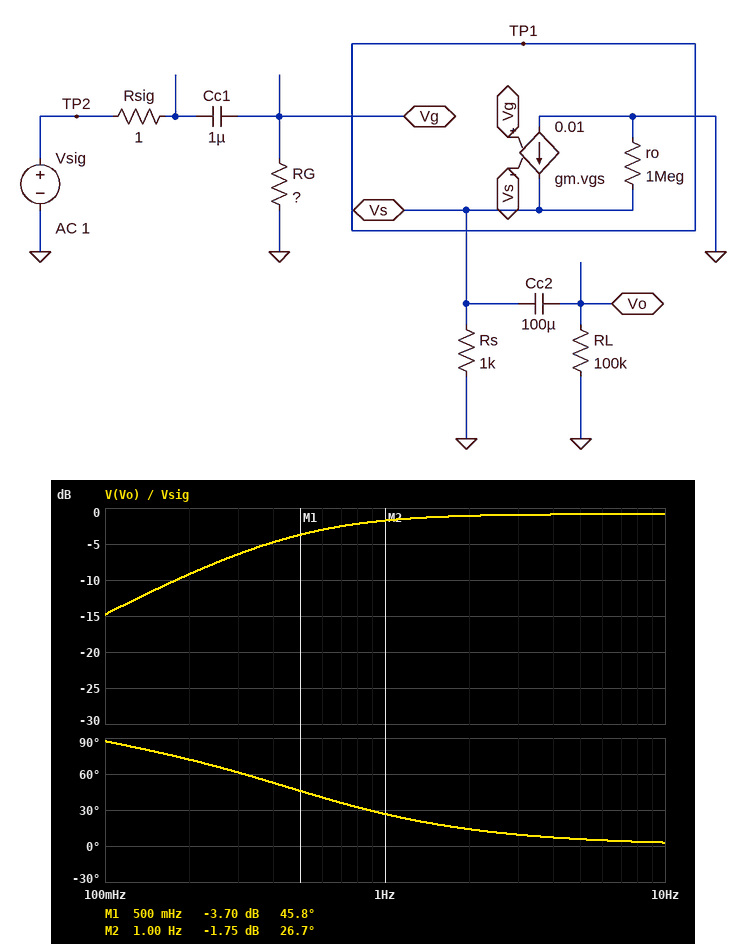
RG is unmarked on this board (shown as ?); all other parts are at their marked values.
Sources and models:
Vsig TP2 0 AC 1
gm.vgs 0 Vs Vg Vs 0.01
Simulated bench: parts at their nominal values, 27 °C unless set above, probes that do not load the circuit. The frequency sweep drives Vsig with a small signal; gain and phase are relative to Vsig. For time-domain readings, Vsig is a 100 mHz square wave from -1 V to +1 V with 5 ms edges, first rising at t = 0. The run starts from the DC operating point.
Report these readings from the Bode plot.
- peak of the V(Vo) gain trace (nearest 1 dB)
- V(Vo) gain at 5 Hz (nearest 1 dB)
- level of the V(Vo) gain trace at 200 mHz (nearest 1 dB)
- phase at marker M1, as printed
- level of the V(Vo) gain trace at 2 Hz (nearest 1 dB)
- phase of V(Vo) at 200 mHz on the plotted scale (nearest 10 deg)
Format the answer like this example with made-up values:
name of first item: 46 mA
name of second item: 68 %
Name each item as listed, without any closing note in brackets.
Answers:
peak of the V(Vo) gain trace: -1 dB
V(Vo) gain at 5 Hz: -1 dB
level of the V(Vo) gain trace at 200 mHz: -9 dB
phase at marker M1, as printed: 45.8 deg
level of the V(Vo) gain trace at 2 Hz: -1 dB
phase of V(Vo) at 200 mHz on the plotted scale: 70 deg
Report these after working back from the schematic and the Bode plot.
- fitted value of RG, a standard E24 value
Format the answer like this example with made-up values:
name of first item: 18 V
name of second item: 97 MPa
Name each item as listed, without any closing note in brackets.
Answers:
fitted value of RG, a standard E24 value: 330 kΩ
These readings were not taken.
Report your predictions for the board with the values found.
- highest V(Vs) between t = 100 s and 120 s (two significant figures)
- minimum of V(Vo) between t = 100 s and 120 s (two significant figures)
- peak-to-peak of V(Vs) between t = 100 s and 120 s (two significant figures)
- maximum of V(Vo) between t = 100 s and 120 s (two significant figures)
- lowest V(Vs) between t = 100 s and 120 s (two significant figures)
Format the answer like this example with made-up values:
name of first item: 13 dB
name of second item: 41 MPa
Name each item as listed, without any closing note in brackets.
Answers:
highest V(Vs) between t = 100 s and 120 s: 1.8 V
minimum of V(Vo) between t = 100 s and 120 s: -1.8 V
peak-to-peak of V(Vs) between t = 100 s and 120 s: 3.6 V
maximum of V(Vo) between t = 100 s and 120 s: 1.8 V
lowest V(Vs) between t = 100 s and 120 s: -1.8 V
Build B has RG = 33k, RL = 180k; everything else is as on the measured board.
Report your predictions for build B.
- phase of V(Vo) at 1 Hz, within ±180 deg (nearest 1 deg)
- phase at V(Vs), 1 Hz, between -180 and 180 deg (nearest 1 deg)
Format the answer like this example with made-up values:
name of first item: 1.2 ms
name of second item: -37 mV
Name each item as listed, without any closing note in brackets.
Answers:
phase of V(Vo) at 1 Hz, within ±180 deg: 79 deg
phase at V(Vs), 1 Hz, between -180 and 180 deg: 78 deg
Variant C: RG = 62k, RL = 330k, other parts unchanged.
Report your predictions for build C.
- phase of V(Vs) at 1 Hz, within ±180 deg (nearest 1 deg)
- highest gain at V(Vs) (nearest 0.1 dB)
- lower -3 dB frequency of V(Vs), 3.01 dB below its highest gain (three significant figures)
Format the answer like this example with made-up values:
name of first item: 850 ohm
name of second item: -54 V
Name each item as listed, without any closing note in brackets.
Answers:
phase of V(Vs) at 1 Hz, within ±180 deg: 69 deg
highest gain at V(Vs): -0.8 dB
lower -3 dB frequency of V(Vs), 3.01 dB below its highest gain: 2.57 Hz
